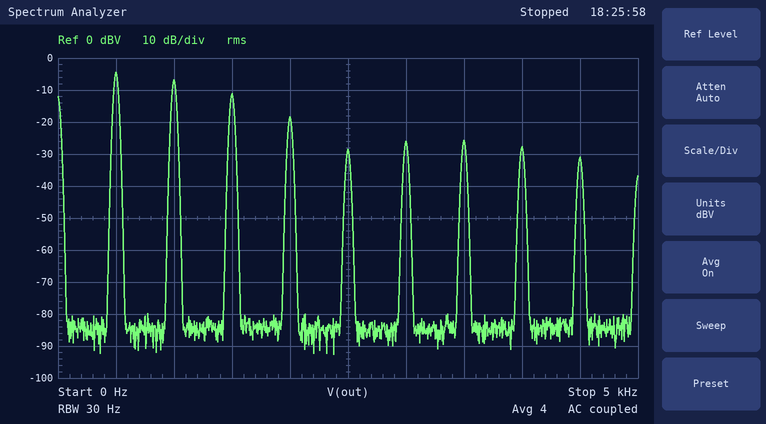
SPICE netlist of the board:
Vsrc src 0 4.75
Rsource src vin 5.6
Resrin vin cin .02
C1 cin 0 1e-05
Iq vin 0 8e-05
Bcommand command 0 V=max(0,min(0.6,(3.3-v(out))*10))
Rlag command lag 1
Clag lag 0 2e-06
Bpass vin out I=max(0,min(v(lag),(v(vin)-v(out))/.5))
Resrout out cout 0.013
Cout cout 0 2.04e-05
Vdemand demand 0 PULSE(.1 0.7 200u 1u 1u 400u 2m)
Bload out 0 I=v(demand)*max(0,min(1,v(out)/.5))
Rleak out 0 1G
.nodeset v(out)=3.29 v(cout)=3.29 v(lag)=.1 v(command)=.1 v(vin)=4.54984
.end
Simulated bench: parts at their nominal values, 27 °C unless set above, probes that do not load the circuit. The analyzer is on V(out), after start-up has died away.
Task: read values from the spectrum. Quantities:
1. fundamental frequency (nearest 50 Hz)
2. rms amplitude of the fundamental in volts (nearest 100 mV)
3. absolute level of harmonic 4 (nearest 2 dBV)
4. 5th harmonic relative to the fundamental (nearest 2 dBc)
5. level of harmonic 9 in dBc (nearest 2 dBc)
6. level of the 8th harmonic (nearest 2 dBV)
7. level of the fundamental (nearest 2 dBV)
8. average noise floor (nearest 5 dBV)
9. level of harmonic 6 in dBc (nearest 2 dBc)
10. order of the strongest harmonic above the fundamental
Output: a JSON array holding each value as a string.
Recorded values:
["500 Hz", "600 mV", "-18 dBV", "-24 dBc", "-26 dBc", "-28 dBV", "-4 dBV", "-85 dBV", "-22 dBc", "2"]
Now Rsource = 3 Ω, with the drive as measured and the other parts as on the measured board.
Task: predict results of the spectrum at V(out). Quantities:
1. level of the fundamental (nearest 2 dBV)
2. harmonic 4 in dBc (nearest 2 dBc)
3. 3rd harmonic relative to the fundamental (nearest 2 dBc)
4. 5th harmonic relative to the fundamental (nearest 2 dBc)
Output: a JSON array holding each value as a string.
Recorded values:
["-10 dBV", "-8 dBc", "-4 dBc", "-12 dBc"]
